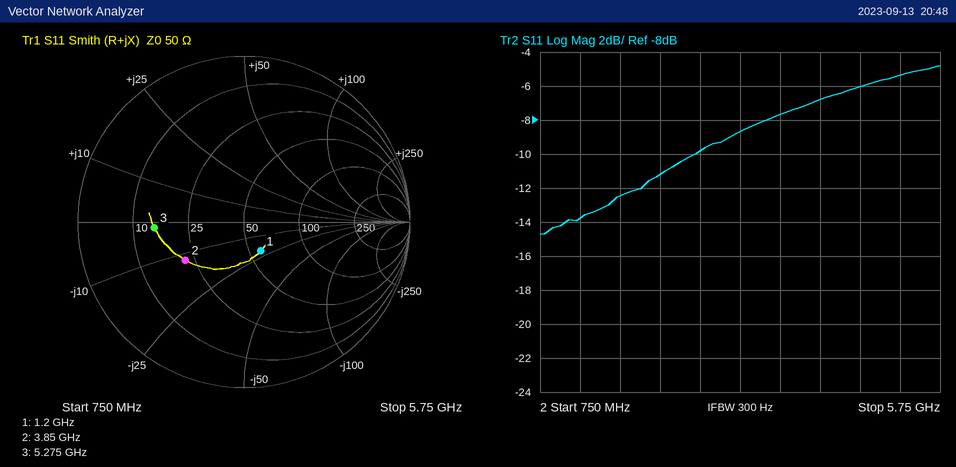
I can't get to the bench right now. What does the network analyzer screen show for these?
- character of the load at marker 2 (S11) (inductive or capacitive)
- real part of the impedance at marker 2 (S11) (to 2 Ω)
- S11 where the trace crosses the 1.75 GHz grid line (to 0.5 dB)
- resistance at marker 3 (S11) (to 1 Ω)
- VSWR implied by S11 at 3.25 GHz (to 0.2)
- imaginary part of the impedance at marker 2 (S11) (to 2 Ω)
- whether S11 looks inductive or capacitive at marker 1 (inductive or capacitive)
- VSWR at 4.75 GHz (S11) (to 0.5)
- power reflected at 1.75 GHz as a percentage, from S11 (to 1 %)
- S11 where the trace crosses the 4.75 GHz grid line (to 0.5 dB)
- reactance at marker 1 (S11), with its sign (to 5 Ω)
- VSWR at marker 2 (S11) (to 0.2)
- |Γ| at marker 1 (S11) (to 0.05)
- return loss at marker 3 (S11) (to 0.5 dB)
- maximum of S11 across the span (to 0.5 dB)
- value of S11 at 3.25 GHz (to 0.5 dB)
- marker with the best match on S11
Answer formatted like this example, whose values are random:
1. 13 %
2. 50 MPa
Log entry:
1. capacitive
2. 22 Ω
3. -12.5 dB
4. 15 Ω
5. 2.2
6. -12 Ω
7. capacitive
8. 3.0
9. 6 %
10. -6.0 dB
11. -20 Ω
12. 2.4
13. 0.20
14. 5.5 dB
15. -5.0 dB
16. -8.5 dB
17. marker 1
